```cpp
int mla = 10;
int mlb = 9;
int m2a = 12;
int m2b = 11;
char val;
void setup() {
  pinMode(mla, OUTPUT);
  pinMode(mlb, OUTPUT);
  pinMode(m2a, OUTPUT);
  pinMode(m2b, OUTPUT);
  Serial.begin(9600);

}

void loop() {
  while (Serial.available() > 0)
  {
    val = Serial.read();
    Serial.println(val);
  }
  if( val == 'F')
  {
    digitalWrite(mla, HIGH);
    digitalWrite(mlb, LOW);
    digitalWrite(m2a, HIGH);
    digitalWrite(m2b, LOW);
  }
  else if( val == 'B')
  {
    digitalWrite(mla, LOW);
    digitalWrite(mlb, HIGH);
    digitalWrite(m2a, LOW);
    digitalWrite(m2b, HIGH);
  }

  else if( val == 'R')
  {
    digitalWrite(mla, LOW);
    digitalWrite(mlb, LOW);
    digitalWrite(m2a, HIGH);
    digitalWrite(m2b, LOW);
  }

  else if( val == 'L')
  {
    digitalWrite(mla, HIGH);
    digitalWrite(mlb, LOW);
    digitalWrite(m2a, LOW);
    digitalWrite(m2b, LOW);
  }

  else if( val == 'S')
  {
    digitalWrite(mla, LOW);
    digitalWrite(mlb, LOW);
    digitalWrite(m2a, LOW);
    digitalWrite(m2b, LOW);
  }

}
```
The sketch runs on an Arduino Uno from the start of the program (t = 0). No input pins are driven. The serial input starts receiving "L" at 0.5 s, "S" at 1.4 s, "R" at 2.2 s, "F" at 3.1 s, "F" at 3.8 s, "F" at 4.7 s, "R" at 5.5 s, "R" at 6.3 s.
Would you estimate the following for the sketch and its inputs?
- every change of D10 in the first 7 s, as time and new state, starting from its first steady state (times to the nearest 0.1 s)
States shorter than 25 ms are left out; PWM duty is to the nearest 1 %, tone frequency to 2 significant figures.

0 s low; 0.5 s high; 1.4 s low; 3.1 s high; 5.5 s low
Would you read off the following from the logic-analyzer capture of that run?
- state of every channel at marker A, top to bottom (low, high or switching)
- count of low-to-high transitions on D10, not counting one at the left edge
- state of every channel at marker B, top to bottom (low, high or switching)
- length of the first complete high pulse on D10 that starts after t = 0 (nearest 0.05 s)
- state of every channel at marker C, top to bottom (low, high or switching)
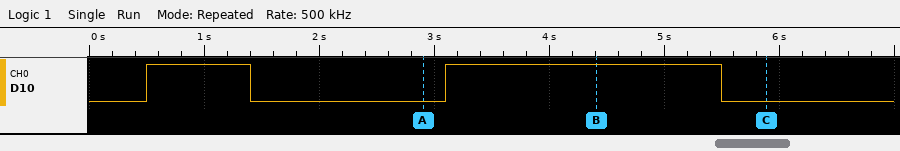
D10 low
2
D10 high
0.90 s
D10 low
